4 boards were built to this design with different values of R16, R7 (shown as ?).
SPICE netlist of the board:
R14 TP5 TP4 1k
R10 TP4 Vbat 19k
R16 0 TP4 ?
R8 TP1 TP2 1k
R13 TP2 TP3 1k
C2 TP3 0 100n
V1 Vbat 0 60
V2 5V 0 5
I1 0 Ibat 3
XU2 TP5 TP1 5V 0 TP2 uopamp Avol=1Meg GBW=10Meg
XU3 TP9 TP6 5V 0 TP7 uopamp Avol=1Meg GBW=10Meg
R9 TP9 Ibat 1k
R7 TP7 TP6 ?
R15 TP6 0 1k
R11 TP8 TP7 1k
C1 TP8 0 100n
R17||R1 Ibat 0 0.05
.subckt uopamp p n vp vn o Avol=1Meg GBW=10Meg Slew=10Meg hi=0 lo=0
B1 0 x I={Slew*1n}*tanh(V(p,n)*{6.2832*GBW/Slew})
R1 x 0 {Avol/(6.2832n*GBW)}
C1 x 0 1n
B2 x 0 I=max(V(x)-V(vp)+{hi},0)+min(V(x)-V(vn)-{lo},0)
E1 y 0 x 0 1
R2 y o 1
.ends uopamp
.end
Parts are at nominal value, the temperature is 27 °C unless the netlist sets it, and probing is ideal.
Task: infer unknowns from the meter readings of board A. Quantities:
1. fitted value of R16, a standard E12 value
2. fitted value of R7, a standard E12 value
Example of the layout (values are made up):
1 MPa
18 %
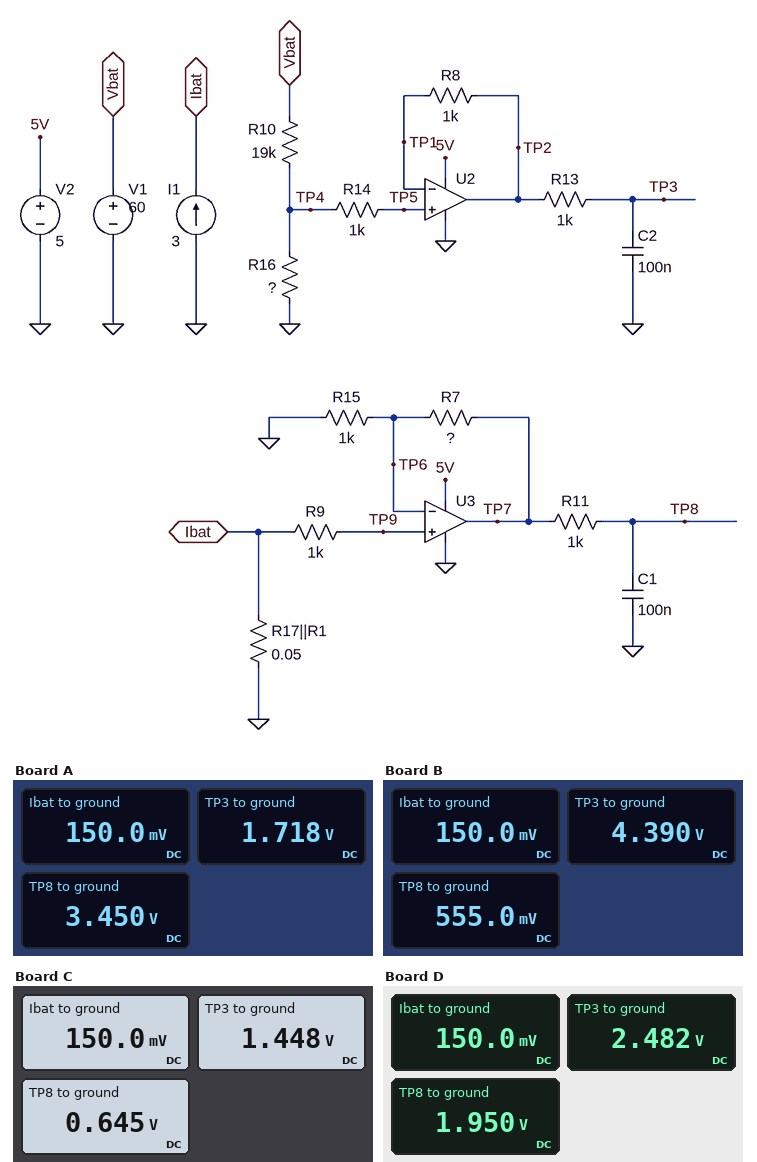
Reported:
560 Ω
22 kΩ
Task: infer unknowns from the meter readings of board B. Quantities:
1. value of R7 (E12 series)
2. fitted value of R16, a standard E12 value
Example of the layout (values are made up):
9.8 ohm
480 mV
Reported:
2.7 kΩ
1.5 kΩ
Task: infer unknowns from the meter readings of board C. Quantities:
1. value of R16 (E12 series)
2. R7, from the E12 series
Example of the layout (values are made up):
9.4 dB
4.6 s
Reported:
470 Ω
3.3 kΩ
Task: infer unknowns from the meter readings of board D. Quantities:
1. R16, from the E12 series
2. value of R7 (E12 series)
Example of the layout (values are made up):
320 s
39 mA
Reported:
820 Ω
12 kΩ
